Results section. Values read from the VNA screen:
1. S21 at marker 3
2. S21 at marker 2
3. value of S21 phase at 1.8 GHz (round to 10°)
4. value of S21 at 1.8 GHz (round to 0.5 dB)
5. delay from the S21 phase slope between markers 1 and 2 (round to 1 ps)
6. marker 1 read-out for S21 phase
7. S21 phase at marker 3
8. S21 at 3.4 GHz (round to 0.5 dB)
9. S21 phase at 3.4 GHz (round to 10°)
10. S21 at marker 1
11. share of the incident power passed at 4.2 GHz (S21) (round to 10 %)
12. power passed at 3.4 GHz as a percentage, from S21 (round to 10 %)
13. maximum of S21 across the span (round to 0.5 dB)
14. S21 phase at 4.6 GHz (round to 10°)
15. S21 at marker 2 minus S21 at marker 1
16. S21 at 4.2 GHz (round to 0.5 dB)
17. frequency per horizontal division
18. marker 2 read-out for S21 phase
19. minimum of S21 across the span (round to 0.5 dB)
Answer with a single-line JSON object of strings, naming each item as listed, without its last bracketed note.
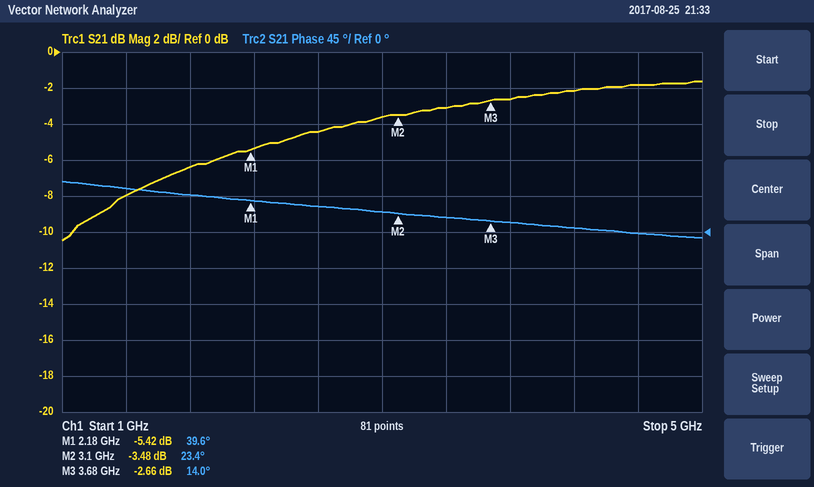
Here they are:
{"S21 at marker 3": "-2.66 dB", "S21 at marker 2": "-3.48 dB", "value of S21 phase at 1.8 GHz": "50°", "value of S21 at 1.8 GHz": "-6.5 dB", "delay from the S21 phase slope between markers 1 and 2": "49 ps", "marker 1 read-out for S21 phase": "39.6°", "S21 phase at marker 3": "14.0°", "S21 at 3.4 GHz": "-3.0 dB", "S21 phase at 3.4 GHz": "20°", "S21 at marker 1": "-5.42 dB", "share of the incident power passed at 4.2 GHz (S21)": "60 %", "power passed at 3.4 GHz as a percentage, from S21": "50 %", "maximum of S21 across the span": "-1.5 dB", "S21 phase at 4.6 GHz": "0°", "S21 at marker 2 minus S21 at marker 1": "1.94 dB", "S21 at 4.2 GHz": "-2.0 dB", "frequency per horizontal division": "400 MHz", "marker 2 read-out for S21 phase": "23.4°", "minimum of S21 across the span": "-10.5 dB"}
